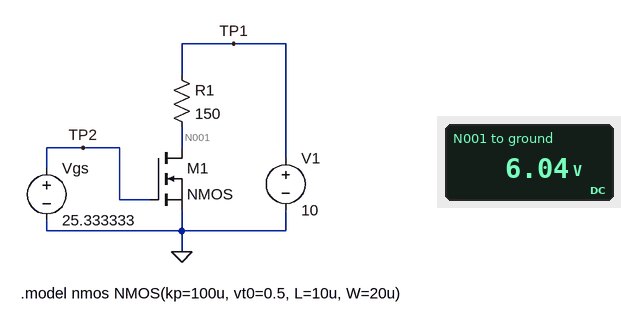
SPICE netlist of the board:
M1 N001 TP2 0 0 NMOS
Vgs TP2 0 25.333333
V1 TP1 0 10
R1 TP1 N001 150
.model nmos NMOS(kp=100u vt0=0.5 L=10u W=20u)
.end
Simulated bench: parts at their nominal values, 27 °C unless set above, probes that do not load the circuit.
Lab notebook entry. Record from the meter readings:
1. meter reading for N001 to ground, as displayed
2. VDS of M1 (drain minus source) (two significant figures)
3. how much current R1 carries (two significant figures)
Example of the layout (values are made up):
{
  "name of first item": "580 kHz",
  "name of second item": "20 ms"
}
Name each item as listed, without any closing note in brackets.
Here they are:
{
  "meter reading for N001 to ground, as displayed": "6.04 V",
  "VDS of M1 (drain minus source)": "6.0 V",
  "how much current R1 carries": "26 mA"
}
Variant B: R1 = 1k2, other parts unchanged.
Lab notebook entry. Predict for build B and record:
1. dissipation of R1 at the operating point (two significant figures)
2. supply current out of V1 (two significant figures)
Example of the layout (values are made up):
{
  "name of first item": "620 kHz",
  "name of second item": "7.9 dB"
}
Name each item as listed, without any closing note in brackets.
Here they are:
{
  "dissipation of R1 at the operating point": "61 mW",
  "supply current out of V1": "7.1 mA"
}
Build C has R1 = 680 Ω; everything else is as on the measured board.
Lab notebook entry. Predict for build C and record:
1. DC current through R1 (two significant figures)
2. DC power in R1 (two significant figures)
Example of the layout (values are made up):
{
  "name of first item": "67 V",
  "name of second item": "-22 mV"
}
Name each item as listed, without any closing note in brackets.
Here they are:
{
  "DC current through R1": "11 mA",
  "DC power in R1": "86 mW"
}
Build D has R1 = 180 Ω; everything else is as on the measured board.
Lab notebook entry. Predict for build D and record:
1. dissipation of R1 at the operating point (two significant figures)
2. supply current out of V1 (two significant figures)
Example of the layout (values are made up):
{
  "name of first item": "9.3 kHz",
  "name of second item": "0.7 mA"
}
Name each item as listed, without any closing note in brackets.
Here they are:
{
  "dissipation of R1 at the operating point": "110 mW",
  "supply current out of V1": "25 mA"
}
